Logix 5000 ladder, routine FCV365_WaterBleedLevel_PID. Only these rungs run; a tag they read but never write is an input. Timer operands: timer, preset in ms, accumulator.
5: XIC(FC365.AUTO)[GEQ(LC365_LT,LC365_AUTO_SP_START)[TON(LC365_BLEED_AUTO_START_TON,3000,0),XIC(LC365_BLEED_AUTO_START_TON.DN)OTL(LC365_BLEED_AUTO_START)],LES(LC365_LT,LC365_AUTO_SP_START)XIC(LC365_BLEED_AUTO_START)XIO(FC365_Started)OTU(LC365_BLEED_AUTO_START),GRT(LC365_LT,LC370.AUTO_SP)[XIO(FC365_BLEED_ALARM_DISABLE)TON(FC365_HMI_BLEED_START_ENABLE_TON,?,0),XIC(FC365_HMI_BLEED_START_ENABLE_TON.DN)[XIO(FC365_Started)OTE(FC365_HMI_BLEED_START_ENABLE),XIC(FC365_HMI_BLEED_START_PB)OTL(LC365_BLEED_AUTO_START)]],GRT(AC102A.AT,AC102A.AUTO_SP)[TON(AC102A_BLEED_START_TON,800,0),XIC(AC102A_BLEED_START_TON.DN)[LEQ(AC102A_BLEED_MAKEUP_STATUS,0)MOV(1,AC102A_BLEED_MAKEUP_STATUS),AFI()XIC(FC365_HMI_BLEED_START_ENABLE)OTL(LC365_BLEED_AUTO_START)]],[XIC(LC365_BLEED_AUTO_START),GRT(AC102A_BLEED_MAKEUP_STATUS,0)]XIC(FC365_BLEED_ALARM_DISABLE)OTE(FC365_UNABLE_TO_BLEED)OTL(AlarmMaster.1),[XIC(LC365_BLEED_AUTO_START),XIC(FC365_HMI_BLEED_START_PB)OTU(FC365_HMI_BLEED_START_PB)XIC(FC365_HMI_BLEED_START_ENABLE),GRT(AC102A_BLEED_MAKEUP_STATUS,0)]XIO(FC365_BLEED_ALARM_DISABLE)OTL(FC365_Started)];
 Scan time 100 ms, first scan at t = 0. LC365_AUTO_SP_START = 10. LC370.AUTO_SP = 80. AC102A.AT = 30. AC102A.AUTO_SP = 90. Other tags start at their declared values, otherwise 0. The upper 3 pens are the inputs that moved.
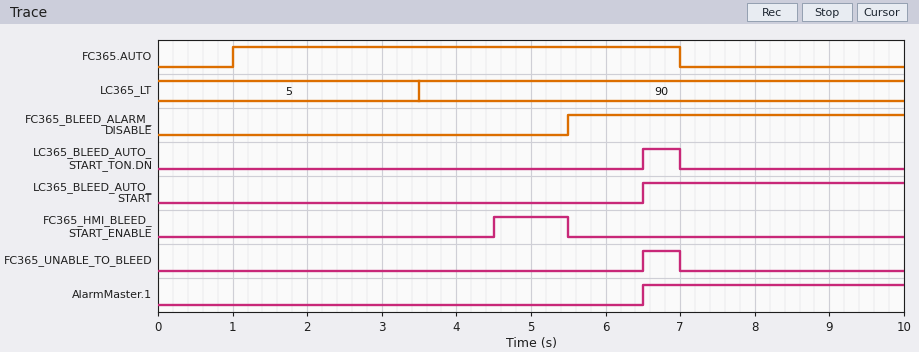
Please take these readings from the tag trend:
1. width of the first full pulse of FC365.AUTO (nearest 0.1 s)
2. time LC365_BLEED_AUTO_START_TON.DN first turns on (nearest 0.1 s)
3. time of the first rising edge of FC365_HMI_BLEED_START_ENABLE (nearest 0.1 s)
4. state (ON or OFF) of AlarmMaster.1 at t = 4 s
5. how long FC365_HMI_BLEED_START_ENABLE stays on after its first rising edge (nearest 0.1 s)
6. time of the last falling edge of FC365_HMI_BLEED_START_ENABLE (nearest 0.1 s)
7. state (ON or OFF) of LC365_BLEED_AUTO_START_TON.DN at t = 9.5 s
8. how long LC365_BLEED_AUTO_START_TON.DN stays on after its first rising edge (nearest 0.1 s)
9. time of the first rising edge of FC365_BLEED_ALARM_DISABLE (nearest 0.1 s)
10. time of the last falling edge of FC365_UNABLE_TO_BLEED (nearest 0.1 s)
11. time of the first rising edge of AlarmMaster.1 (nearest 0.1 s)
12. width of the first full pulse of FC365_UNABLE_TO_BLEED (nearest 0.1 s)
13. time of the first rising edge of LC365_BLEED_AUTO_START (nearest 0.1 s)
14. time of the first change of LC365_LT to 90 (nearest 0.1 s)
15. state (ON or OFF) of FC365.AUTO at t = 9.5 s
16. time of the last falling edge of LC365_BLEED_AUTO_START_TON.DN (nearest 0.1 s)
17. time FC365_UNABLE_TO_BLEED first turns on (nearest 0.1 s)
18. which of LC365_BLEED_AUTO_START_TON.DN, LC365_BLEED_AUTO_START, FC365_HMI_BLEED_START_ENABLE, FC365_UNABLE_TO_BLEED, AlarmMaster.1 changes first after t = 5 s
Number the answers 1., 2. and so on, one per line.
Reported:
1. 6.0 s
2. 6.5 s
3. 4.5 s
4. OFF
5. 1.0 s
6. 5.5 s
7. OFF
8. 0.5 s
9. 5.5 s
10. 7.0 s
11. 6.5 s
12. 0.5 s
13. 6.5 s
14. 3.5 s
15. OFF
16. 7.0 s
17. 6.5 s
18. FC365_HMI_BLEED_START_ENABLE
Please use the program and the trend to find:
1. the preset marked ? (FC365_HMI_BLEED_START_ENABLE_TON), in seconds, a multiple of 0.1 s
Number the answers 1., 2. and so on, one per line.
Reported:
1. 1.0 s
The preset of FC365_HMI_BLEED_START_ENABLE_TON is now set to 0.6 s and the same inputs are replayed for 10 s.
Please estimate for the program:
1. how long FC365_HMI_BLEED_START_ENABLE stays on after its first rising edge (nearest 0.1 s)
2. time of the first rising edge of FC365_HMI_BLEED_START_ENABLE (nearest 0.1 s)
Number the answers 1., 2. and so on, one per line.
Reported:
1. 1.4 s
2. 4.1 s
